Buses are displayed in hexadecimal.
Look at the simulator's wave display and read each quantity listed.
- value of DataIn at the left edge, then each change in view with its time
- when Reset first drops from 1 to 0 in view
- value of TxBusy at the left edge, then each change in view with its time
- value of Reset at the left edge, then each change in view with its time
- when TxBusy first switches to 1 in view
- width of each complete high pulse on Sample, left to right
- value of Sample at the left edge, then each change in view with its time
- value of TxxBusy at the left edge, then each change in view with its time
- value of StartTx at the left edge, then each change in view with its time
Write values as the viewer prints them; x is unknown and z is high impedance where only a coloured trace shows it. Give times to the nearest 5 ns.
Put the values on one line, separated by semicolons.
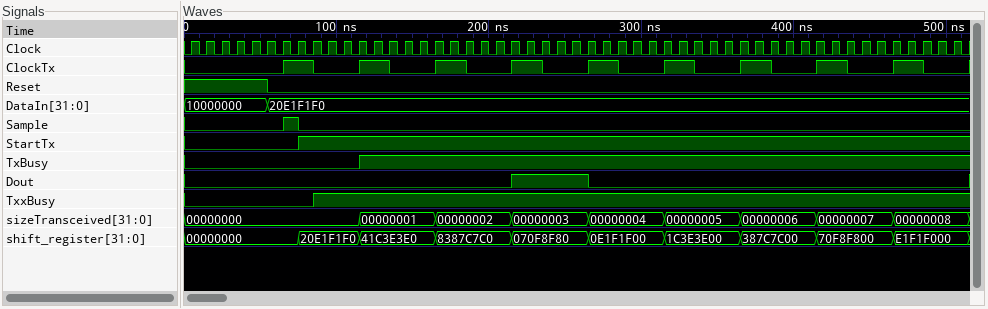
10000000, 20E1F1F0 at 55 ns; 55 ns; 0, 1 at 115 ns; 1, 0 at 55 ns; 115 ns; 10 ns; 0, 1 at 65 ns, 0 at 75 ns; 0, 1 at 85 ns; 0, 1 at 75 ns
